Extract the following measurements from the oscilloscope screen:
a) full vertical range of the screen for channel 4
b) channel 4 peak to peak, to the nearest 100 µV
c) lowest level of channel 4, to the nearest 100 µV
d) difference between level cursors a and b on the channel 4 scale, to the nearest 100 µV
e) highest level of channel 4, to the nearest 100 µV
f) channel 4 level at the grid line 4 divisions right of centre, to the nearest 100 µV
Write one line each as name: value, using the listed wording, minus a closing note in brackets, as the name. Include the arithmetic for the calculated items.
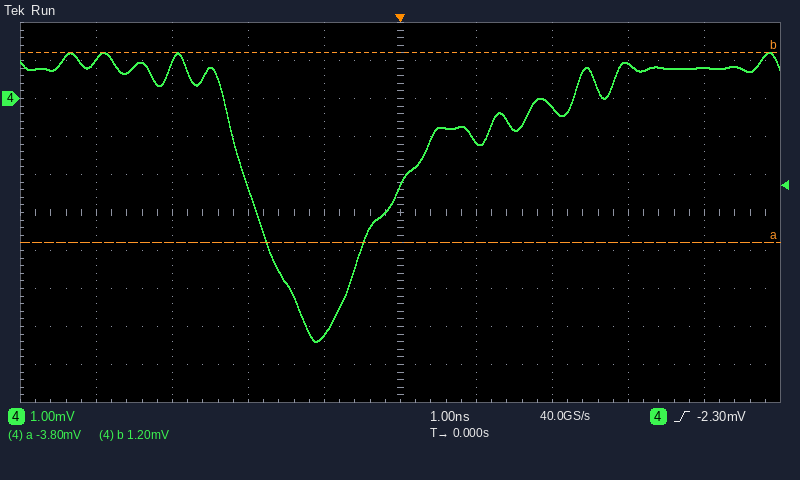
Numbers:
full vertical range of the screen for channel 4: 10 mV
channel 4 peak to peak, to the nearest 100 µV: 1.2 mV − (-6.4 mV) = 7.6 mV
lowest level of channel 4, to the nearest 100 µV: -6.4 mV
difference between level cursors a and b on the channel 4 scale, to the nearest 100 µV: 5.0 mV
highest level of channel 4, to the nearest 100 µV: 1.2 mV
channel 4 level at the grid line 4 divisions right of centre, to the nearest 100 µV: 800 µV
